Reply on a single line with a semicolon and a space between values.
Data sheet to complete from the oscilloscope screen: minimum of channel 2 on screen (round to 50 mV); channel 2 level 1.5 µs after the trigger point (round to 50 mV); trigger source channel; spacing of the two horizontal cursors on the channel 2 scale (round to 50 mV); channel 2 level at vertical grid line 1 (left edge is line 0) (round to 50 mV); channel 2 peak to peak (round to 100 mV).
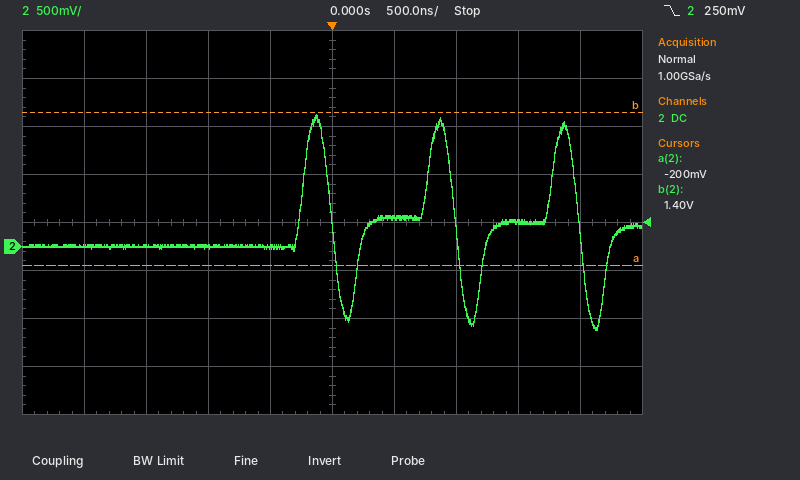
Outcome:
-850 mV; 250 mV; channel 2; 1.60 V; 0 mV; 2.20 V
